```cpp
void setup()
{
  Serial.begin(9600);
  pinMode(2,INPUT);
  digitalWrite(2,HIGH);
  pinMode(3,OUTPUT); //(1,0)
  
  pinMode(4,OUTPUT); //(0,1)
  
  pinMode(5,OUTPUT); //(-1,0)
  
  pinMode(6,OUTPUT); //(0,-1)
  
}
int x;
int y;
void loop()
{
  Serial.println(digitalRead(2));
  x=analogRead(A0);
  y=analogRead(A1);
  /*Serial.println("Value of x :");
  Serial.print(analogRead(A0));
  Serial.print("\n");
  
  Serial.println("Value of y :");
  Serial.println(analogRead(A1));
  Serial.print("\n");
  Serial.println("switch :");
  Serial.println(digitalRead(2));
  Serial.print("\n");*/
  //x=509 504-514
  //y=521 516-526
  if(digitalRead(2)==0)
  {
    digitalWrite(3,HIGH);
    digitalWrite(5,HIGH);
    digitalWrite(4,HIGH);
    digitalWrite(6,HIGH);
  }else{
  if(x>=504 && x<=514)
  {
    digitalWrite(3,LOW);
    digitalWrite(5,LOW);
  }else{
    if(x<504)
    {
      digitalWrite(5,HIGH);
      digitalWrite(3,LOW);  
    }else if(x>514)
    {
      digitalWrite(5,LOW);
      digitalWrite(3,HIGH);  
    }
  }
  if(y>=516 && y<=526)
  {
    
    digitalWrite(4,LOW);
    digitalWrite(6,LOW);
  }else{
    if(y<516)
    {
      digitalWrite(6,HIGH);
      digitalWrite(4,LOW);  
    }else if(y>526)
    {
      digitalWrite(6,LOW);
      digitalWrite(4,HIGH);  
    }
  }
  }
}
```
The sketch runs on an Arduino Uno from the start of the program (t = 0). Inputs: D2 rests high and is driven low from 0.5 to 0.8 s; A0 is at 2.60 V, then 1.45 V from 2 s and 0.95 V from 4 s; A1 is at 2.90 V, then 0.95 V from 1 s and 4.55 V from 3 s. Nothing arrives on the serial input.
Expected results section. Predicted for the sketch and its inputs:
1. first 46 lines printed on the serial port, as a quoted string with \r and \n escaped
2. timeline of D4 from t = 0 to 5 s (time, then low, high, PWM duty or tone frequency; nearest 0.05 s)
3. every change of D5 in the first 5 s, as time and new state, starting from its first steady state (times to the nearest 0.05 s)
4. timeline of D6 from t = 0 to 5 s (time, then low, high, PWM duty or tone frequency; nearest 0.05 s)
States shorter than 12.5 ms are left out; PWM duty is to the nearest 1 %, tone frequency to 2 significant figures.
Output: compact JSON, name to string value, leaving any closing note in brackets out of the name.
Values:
{"first 46 lines printed on the serial port, as a quoted string with \\r and \\n escaped": "\"1\\r\\n1\\r\\n1\\r\\n1\\r\\n1\\r\\n1\\r\\n1\\r\\n1\\r\\n1\\r\\n1\\r\\n1\\r\\n1\\r\\n1\\r\\n1\\r\\n1\\r\\n1\\r\\n1\\r\\n1\\r\\n1\\r\\n1\\r\\n1\\r\\n1\\r\\n1\\r\\n1\\r\\n1\\r\\n1\\r\\n1\\r\\n1\\r\\n1\\r\\n1\\r\\n1\\r\\n1\\r\\n1\\r\\n1\\r\\n1\\r\\n1\\r\\n1\\r\\n1\\r\\n1\\r\\n1\\r\\n1\\r\\n1\\r\\n1\\r\\n1\\r\\n1\\r\\n1\\r\\n\"", "timeline of D4 from t = 0 to 5 s": "0 s high; 1 s low; 3 s high", "every change of D5 in the first 5 s, as time and new state, starting from its first steady state": "0 s low; 0.5 s high; 0.8 s low; 2 s high", "timeline of D6 from t = 0 to 5 s": "0 s low; 0.5 s high; 0.8 s low; 1 s high; 3 s low"}
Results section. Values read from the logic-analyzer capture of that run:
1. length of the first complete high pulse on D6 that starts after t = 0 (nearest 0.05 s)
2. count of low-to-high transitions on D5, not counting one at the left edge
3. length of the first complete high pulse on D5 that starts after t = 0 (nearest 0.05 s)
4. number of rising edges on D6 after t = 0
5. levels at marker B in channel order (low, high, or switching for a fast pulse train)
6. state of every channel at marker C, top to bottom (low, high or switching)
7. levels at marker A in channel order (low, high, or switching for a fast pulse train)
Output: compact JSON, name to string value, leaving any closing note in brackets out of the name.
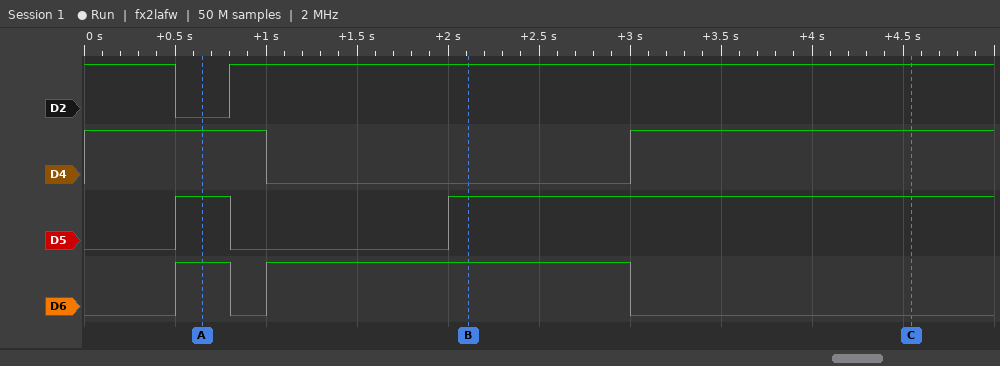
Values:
{"length of the first complete high pulse on D6 that starts after t = 0": "0.30 s", "count of low-to-high transitions on D5, not counting one at the left edge": "2", "length of the first complete high pulse on D5 that starts after t = 0": "0.30 s", "number of rising edges on D6 after t = 0": "2", "levels at marker B in channel order": "D2 high, D4 low, D5 high, D6 high", "state of every channel at marker C, top to bottom": "D2 high, D4 high, D5 high, D6 low", "levels at marker A in channel order": "D2 low, D4 high, D5 high, D6 high"}
